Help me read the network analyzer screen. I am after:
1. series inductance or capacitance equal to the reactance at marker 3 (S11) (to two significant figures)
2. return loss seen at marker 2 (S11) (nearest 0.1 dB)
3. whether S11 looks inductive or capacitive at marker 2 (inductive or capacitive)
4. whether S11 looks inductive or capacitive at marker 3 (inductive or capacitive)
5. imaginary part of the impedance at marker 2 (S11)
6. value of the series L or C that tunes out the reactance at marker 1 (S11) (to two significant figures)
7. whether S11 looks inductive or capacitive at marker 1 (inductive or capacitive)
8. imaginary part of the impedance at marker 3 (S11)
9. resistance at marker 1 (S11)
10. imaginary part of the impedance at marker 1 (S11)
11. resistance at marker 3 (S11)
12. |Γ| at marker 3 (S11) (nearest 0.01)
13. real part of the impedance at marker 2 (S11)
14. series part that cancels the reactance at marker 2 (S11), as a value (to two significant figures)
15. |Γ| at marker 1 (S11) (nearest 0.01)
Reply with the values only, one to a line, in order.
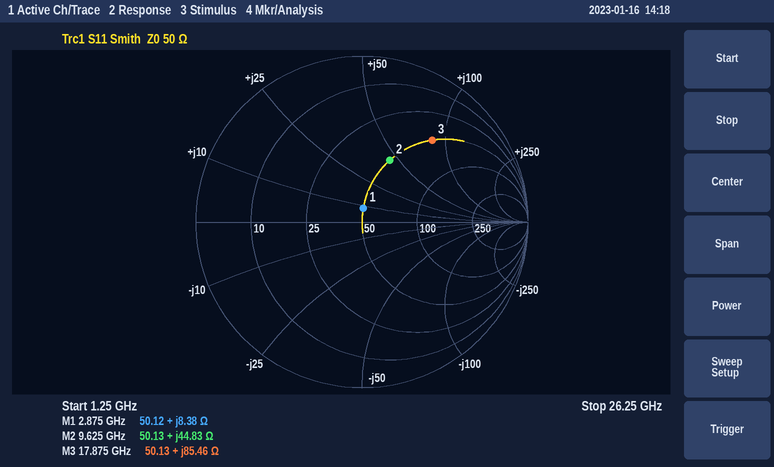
760 pH
7.8 dB
inductive
inductive
+44.83 Ω
6.6 pF
inductive
+85.46 Ω
50.12 Ω
+8.38 Ω
50.13 Ω
0.65
50.13 Ω
370 fF
0.08
